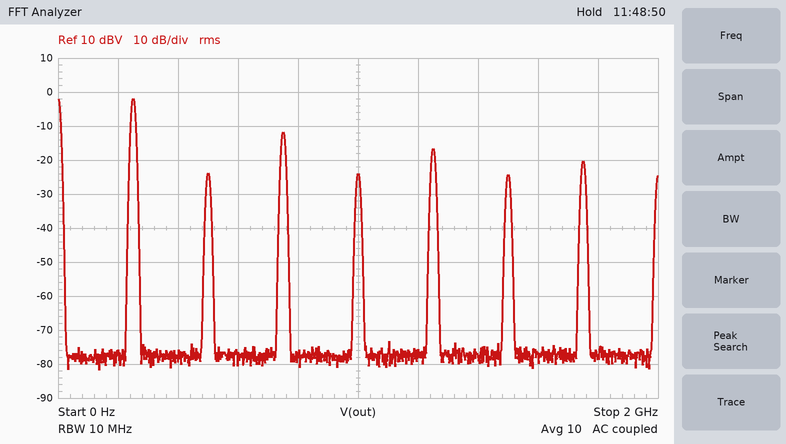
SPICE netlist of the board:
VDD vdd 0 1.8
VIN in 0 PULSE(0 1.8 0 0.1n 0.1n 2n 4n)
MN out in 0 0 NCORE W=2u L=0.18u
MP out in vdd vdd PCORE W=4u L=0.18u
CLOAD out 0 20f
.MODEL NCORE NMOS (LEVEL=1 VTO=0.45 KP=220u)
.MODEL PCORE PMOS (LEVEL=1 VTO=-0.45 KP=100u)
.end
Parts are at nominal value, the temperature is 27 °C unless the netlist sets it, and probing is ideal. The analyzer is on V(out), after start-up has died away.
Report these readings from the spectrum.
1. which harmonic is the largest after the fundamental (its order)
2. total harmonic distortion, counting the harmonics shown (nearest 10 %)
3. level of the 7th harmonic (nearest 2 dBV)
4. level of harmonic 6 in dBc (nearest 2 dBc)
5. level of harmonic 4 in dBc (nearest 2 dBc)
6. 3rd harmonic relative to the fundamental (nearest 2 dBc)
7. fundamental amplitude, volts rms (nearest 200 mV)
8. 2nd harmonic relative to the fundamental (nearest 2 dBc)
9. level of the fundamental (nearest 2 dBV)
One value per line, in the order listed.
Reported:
3
40 %
-20 dBV
-22 dBc
-22 dBc
-10 dBc
800 mV
-22 dBc
-2 dBV
